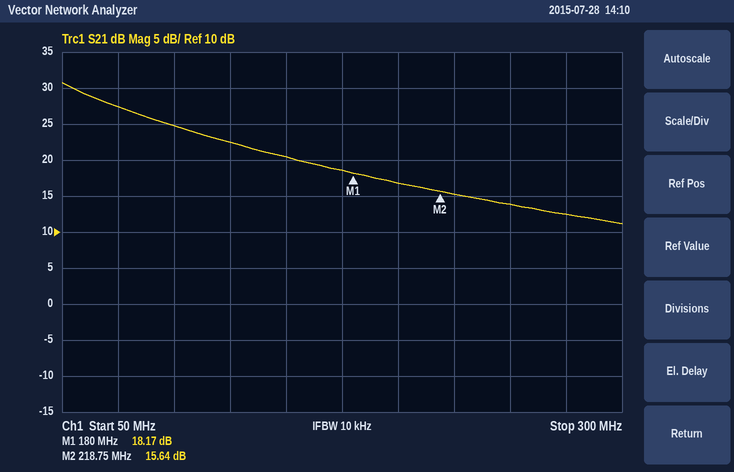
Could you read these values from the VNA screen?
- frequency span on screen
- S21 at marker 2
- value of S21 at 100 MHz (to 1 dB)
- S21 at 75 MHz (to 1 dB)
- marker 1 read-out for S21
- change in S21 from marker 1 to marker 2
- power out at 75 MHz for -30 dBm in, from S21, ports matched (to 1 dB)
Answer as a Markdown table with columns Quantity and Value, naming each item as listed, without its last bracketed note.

| Quantity | Value |
|---|---|
| frequency span on screen | 250 MHz |
| S21 at marker 2 | 15.64 dB |
| value of S21 at 100 MHz | 25 dB |
| S21 at 75 MHz | 27 dB |
| marker 1 read-out for S21 | 18.17 dB |
| change in S21 from marker 1 to marker 2 | -2.53 dB |
| power out at 75 MHz for -30 dBm in, from S21, ports matched | -3 dBm |
